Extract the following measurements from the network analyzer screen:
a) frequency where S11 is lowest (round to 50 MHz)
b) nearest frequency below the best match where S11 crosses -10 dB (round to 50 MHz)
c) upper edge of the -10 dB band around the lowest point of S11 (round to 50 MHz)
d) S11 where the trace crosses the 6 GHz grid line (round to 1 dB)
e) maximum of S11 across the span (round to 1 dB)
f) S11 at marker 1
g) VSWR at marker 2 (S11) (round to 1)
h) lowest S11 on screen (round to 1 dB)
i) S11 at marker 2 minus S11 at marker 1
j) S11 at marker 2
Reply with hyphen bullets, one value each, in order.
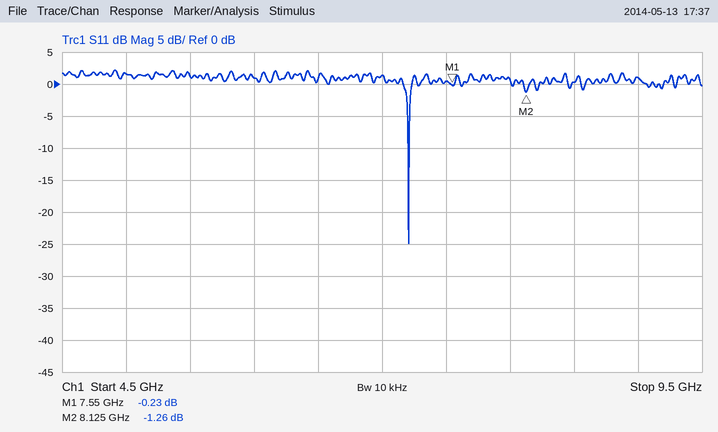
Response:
- 7.20 GHz
- 7.20 GHz
- 7.20 GHz
- 1 dB
- 2 dB
- -0.23 dB
- 14
- -25 dB
- -1.03 dB
- -1.26 dB
